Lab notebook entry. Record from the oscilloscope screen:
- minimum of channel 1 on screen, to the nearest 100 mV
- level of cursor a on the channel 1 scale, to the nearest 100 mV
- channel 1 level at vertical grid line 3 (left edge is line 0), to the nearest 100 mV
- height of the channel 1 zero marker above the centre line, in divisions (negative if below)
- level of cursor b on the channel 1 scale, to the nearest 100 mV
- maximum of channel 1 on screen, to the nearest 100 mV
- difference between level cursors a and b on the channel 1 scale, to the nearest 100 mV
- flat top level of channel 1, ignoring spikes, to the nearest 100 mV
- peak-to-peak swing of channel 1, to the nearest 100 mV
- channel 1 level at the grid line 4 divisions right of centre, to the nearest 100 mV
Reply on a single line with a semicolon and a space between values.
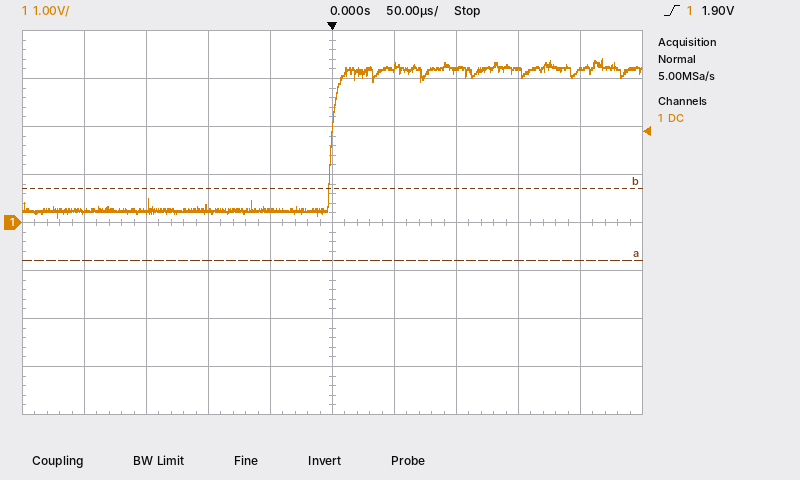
100 mV; -800 mV; 300 mV; 0.0 div; 700 mV; 3.4 V; 1.5 V; 3.2 V; 3.3 V; 3.2 V
